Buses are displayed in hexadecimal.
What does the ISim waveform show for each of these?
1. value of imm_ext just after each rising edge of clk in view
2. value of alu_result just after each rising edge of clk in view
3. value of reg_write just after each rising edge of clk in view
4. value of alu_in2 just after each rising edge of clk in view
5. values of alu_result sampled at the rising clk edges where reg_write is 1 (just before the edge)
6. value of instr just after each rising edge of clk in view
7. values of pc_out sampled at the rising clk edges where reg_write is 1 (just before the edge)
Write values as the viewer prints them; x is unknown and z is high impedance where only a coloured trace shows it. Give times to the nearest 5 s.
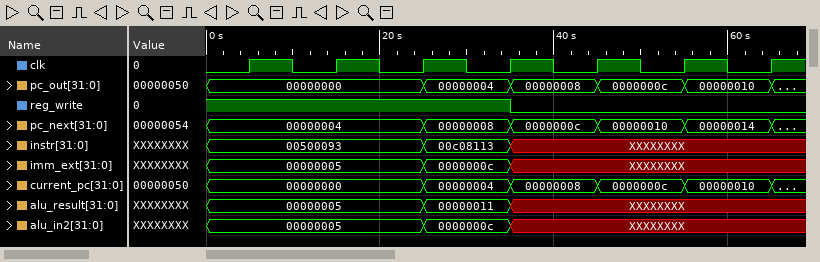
00000005, 00000005, 0000000c, XXXXXXXX, XXXXXXXX, XXXXXXXX, XXXXXXXX
00000005, 00000005, 00000011, XXXXXXXX, XXXXXXXX, XXXXXXXX, XXXXXXXX
1 1 1 0 0 0 0
00000005, 00000005, 0000000c, XXXXXXXX, XXXXXXXX, XXXXXXXX, XXXXXXXX
00000005, 00000005, 00000005, 00000011
00500093, 00500093, 00c08113, XXXXXXXX, XXXXXXXX, XXXXXXXX, XXXXXXXX
00000000, 00000000, 00000000, 00000004
